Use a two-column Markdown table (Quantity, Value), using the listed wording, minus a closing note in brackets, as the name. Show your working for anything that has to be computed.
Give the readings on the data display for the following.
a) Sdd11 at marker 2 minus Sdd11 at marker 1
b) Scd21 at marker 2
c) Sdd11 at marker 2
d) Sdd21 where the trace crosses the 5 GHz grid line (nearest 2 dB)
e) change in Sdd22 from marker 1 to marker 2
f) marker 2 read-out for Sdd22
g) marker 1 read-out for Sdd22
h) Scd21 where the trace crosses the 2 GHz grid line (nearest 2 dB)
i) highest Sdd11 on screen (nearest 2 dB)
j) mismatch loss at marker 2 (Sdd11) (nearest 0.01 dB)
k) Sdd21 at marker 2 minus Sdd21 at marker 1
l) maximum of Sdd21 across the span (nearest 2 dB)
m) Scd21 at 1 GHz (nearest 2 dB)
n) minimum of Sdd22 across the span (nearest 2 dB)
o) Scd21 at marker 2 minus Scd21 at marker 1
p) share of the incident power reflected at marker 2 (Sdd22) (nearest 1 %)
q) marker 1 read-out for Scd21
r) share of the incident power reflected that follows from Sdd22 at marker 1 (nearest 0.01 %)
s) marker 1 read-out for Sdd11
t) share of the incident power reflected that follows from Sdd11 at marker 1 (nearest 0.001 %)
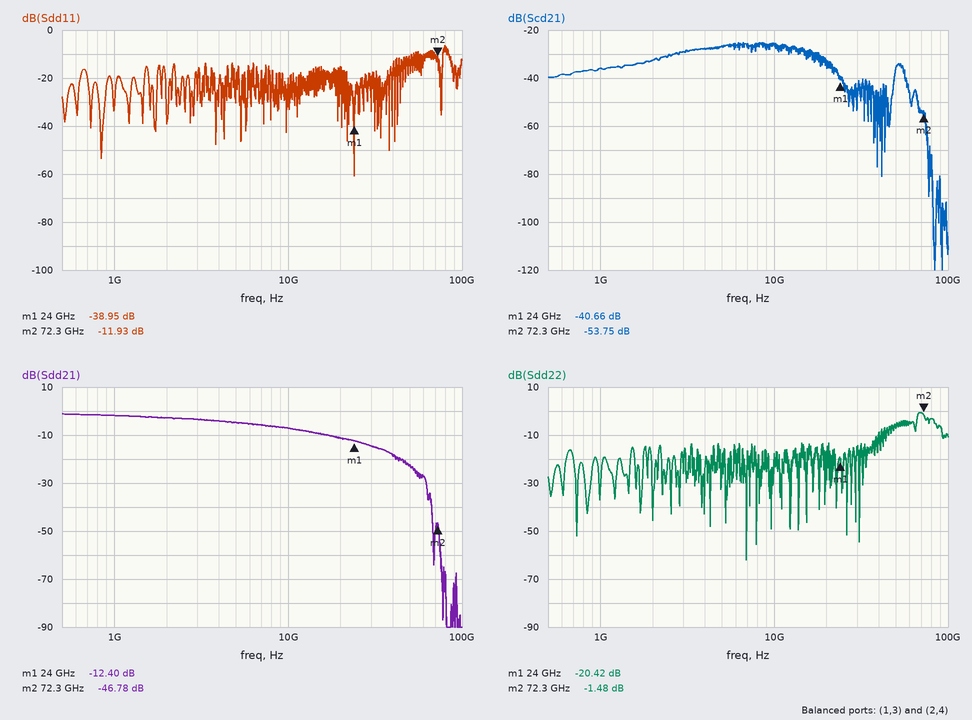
| Quantity | Value |
|---|---|
| Sdd11 at marker 2 minus Sdd11 at marker 1 | -11.93 − (-38.95) = 27.02 dB |
| Scd21 at marker 2 | -53.75 dB |
| Sdd11 at marker 2 | -11.93 dB |
| Sdd21 where the trace crosses the 5 GHz grid line | -4 dB |
| change in Sdd22 from marker 1 to marker 2 | -1.48 − (-20.42) = 18.94 dB |
| marker 2 read-out for Sdd22 | -1.48 dB |
| marker 1 read-out for Sdd22 | -20.42 dB |
| Scd21 where the trace crosses the 2 GHz grid line | -32 dB |
| highest Sdd11 on screen | -6 dB |
| mismatch loss at marker 2 (Sdd11) | −10 log10(1 − 10^(-11.93/10)) ≈ 0.29 dB |
| Sdd21 at marker 2 minus Sdd21 at marker 1 | -46.78 − (-12.4) = -34.38 dB |
| maximum of Sdd21 across the span | -2 dB |
| Scd21 at 1 GHz | -36 dB |
| minimum of Sdd22 across the span | -62 dB |
| Scd21 at marker 2 minus Scd21 at marker 1 | -53.75 − (-40.66) = -13.09 dB |
| share of the incident power reflected at marker 2 (Sdd22) | 10^(-1.48/10) ≈ 71 % |
| marker 1 read-out for Scd21 | -40.66 dB |
| share of the incident power reflected that follows from Sdd22 at marker 1 | 10^(-20.42/10) ≈ 0.91 % |
| marker 1 read-out for Sdd11 | -38.95 dB |
| share of the incident power reflected that follows from Sdd11 at marker 1 | 10^(-38.95/10) ≈ 0.013 % |
